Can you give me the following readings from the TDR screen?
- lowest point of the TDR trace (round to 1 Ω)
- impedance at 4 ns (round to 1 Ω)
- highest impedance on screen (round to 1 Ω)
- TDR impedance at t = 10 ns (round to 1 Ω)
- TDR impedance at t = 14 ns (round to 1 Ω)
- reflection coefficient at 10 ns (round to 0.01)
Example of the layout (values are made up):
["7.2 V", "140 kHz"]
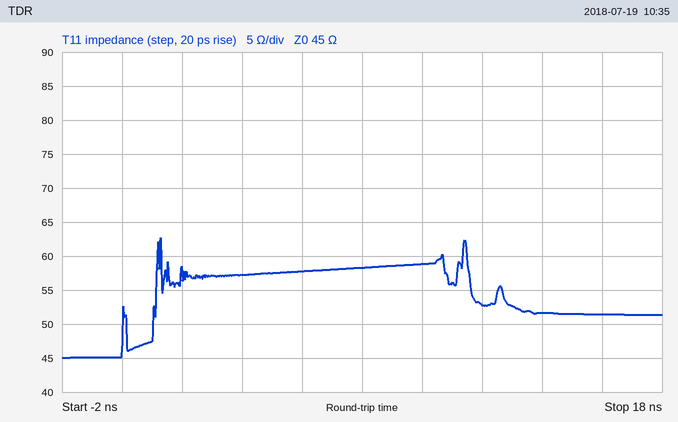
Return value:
["45 Ω", "57 Ω", "63 Ω", "59 Ω", "52 Ω", "+0.13"]
